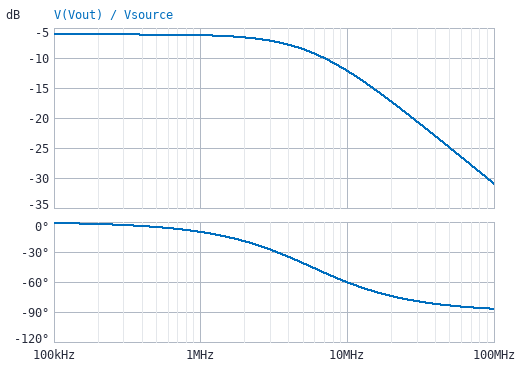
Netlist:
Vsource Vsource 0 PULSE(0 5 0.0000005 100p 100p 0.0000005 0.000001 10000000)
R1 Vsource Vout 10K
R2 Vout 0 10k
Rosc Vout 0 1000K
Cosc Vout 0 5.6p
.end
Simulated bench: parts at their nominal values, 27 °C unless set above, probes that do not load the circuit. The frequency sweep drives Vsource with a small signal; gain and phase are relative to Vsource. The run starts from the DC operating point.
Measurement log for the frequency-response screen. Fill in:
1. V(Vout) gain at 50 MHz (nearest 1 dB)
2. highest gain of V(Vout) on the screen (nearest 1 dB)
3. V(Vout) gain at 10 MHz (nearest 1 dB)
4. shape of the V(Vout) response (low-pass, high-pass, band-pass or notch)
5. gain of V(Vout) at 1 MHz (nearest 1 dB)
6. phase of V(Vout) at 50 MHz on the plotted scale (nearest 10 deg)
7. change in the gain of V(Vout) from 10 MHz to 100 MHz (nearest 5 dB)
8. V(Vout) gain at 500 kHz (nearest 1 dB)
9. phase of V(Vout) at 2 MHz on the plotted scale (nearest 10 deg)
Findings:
-25 dB
-6 dB
-12 dB
low-pass
-6 dB
-80 deg
-20 dB
-6 dB
-20 deg
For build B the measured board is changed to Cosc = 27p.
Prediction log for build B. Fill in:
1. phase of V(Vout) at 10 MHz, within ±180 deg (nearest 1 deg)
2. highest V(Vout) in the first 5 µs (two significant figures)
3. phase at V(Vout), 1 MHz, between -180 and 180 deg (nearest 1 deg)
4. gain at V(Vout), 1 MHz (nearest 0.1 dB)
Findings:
-83 deg
2.4 V
-40 deg
-8.4 dB
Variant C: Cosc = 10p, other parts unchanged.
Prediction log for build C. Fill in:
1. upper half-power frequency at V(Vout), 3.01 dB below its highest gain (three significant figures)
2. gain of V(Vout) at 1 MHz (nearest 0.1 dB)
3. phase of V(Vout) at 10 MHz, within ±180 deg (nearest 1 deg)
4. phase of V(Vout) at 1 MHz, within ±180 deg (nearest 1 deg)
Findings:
3.20 MHz
-6.5 dB
-72 deg
-17 deg
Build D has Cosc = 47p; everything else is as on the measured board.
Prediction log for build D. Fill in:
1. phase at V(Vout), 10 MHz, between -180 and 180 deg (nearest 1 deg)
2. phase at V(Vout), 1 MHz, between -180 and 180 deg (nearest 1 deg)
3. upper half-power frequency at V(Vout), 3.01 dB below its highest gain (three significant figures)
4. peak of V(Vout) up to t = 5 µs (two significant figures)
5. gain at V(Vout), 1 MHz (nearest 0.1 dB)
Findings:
-86 deg
-56 deg
681 kHz
2.2 V
-11.1 dB
